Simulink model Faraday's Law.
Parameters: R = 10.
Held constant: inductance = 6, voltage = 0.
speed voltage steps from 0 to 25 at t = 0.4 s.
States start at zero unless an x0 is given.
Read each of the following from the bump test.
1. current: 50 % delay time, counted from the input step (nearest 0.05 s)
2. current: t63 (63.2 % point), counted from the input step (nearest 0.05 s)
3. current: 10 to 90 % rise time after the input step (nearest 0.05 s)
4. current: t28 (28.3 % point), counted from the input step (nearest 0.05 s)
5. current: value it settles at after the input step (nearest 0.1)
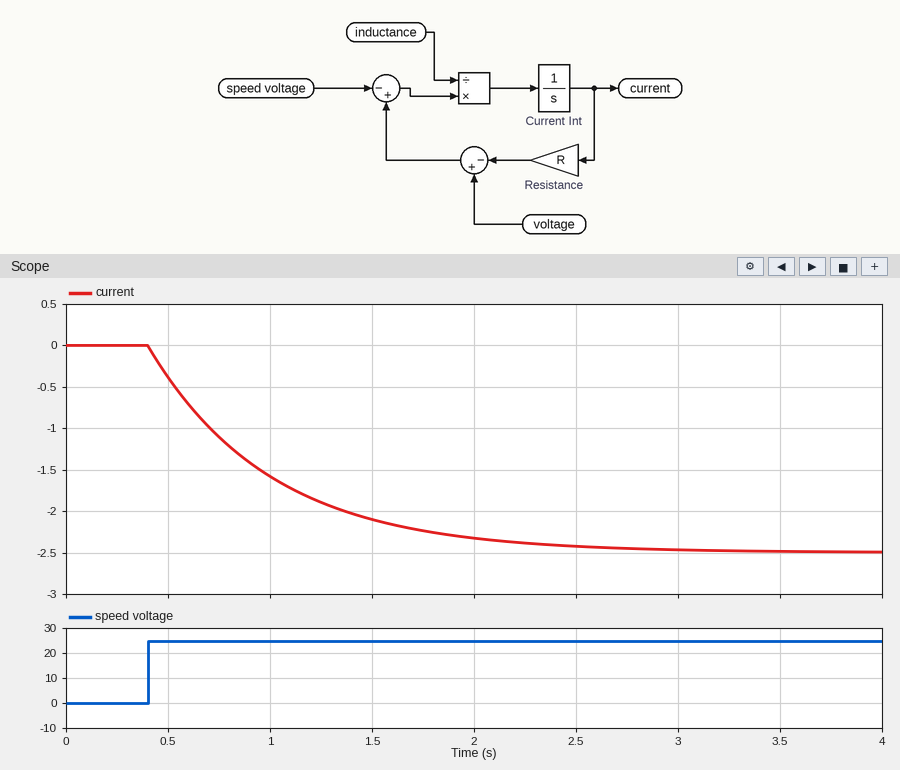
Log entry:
0.40 s
0.60 s
1.30 s
0.20 s
-2.5
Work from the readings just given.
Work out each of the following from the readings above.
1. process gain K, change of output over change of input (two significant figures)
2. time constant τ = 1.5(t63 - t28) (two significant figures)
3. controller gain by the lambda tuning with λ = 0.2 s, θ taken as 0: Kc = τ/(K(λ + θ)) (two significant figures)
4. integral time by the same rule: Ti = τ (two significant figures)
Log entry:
-0.10
0.60 s
-30
0.60 s
